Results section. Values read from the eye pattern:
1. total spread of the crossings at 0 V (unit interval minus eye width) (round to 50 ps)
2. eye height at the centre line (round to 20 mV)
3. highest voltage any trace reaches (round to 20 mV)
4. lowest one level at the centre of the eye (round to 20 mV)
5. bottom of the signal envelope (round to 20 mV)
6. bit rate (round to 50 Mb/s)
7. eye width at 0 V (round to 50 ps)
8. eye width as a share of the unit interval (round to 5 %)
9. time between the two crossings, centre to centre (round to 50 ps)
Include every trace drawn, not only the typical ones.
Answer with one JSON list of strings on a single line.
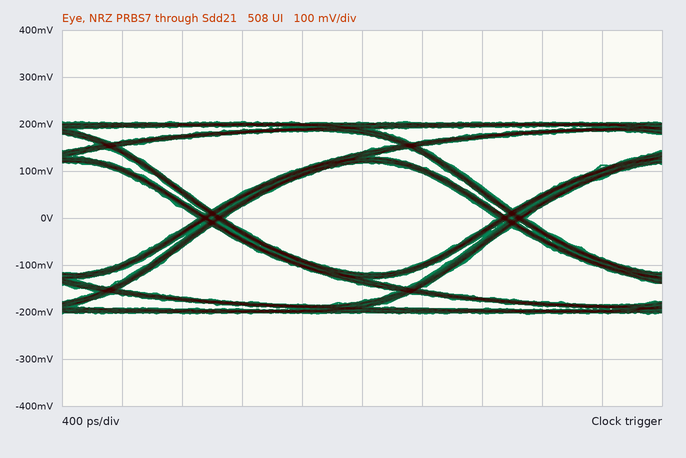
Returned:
["200 ps", "240 mV", "200 mV", "120 mV", "-200 mV", "500 Mb/s", "1.80 ns", "90 %", "2.00 ns"]
